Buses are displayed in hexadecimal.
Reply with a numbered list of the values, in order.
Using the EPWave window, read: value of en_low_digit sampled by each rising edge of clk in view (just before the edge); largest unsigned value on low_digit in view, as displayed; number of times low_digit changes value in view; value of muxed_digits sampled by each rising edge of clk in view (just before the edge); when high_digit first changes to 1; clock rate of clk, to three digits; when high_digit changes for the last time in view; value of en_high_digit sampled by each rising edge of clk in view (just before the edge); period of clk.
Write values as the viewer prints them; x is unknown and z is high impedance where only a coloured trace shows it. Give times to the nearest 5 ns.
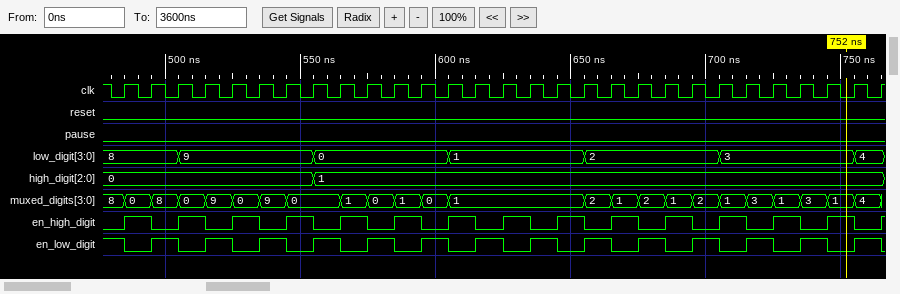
1. 1 0 1 0 1 0 1 0 1 0 1 0 1 0 1 0 1 0 1 0 1 0 1 0 1 0 1 0 1
2. 9
3. 6
4. 8, 0, 8, 0, 9, 0, 9, 0, 0, 1, 0, 1, 0, 1, 1, 1, 1, 1, 2, 1, 2, 1, 2, 1, 3, 1, 3, 1, 4
5. 555 ns
6. 100 MHz
7. 555 ns
8. 0 1 0 1 0 1 0 1 0 1 0 1 0 1 0 1 0 1 0 1 0 1 0 1 0 1 0 1 0
9. 10 ns
